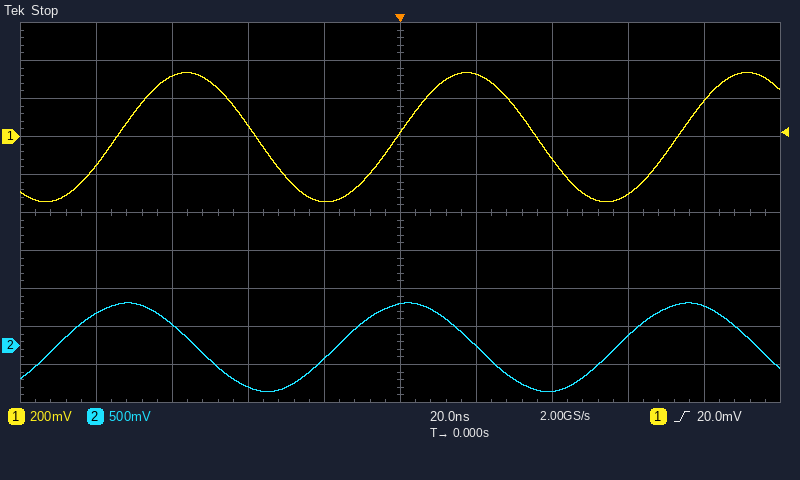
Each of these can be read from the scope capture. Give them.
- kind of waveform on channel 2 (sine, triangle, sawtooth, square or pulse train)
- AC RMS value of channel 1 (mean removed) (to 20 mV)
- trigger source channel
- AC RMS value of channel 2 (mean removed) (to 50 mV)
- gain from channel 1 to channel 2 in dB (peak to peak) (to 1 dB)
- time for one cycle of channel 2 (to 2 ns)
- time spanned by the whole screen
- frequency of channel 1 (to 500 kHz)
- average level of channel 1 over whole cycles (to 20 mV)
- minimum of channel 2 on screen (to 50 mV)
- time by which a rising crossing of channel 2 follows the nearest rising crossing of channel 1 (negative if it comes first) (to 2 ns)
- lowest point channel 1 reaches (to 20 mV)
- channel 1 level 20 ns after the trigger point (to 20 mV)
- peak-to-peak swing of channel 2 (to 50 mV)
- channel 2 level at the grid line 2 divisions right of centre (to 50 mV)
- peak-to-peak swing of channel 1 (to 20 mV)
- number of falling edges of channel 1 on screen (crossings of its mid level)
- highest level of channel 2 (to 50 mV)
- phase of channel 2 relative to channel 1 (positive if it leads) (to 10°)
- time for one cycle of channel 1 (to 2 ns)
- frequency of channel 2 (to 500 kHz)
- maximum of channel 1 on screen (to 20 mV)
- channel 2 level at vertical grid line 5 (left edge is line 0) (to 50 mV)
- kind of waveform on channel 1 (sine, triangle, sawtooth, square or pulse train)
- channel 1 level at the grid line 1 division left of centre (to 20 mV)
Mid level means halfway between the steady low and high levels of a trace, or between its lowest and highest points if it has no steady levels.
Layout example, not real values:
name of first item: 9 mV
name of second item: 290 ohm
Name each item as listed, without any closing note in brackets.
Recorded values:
kind of waveform on channel 2: sine
AC RMS value of channel 1 (mean removed): 240 mV
trigger source channel: channel 1
AC RMS value of channel 2 (mean removed): 400 mV
gain from channel 1 to channel 2 in dB (peak to peak): 5 dB
time for one cycle of channel 2: 74 ns
time spanned by the whole screen: 200 ns
frequency of channel 1: 13.5 MHz
average level of channel 1 over whole cycles: 0 mV
minimum of channel 2 on screen: -600 mV
time by which a rising crossing of channel 2 follows the nearest rising crossing of channel 1 (negative if it comes first): -16 ns
lowest point channel 1 reaches: -340 mV
channel 1 level 20 ns after the trigger point: 320 mV
peak-to-peak swing of channel 2: 1.15 V
channel 2 level at the grid line 2 divisions right of centre: -600 mV
peak-to-peak swing of channel 1: 680 mV
number of falling edges of channel 1 on screen: 2
highest level of channel 2: 550 mV
phase of channel 2 relative to channel 1 (positive if it leads): +80°
time for one cycle of channel 1: 74 ns
frequency of channel 2: 13.5 MHz
maximum of channel 1 on screen: 340 mV
channel 2 level at vertical grid line 5 (left edge is line 0): 550 mV
kind of waveform on channel 1: sine
channel 1 level at the grid line 1 division left of centre: -340 mV
